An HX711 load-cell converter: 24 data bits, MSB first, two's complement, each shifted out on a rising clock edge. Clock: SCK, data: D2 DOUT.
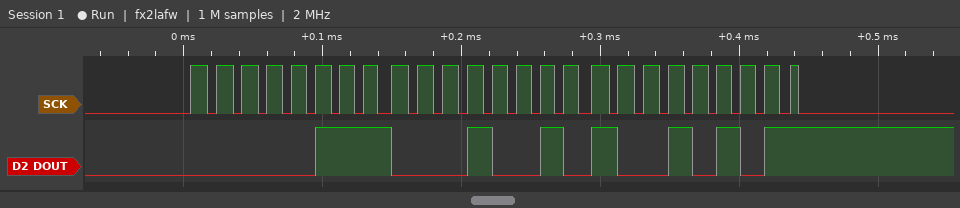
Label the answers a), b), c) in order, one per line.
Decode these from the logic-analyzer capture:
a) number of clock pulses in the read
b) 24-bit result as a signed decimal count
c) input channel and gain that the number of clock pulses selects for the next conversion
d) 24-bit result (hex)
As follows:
a) 25
b) 463509
c) channel A, gain 128
d) 0x071295
